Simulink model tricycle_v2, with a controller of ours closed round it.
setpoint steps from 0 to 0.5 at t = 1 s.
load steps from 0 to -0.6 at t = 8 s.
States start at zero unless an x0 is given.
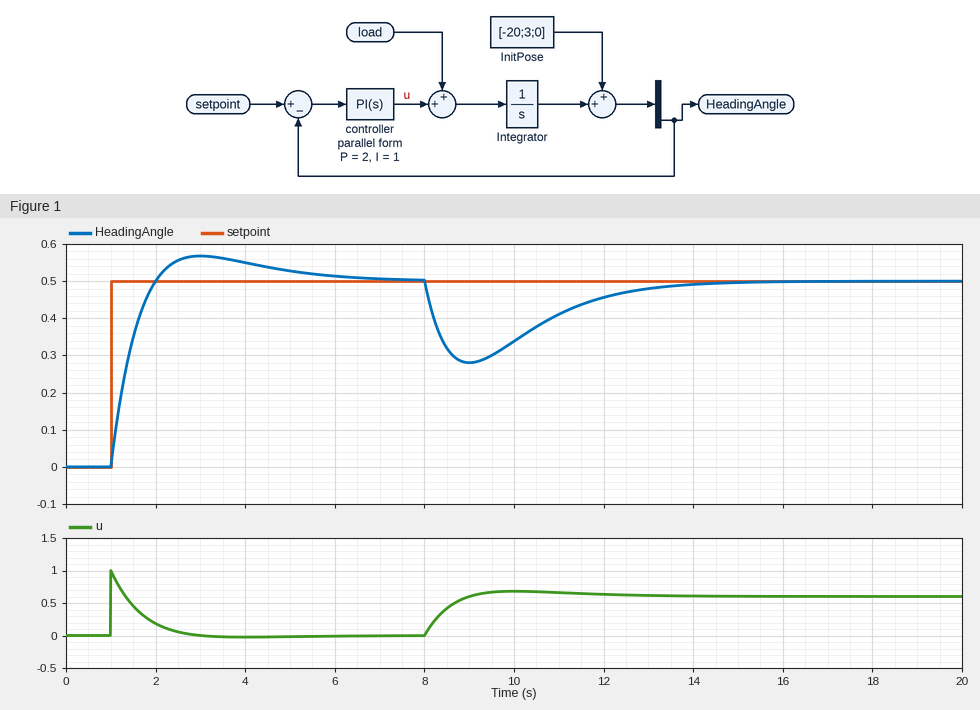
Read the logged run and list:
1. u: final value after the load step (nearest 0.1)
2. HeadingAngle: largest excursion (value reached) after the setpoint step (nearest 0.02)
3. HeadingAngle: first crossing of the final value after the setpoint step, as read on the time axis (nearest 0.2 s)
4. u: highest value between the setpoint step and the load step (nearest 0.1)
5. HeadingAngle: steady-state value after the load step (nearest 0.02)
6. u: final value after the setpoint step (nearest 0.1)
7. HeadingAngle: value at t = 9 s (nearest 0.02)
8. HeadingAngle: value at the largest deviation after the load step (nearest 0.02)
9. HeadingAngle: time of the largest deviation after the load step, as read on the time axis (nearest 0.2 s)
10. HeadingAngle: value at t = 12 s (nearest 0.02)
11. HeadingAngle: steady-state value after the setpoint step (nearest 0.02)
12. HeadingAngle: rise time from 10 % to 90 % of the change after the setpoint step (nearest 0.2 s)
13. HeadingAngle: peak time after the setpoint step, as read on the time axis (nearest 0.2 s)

0.6
0.56
2.0 s
1.0
0.50
0.0
0.28
0.28
9.0 s
0.46
0.50
0.8 s
3.0 s
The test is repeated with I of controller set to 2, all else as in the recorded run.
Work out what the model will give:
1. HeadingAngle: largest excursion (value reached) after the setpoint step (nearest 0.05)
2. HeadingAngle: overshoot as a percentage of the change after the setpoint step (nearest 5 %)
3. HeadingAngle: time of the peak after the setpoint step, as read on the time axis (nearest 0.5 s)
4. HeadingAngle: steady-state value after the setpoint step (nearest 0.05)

0.60
20 %
2.5 s
0.50
